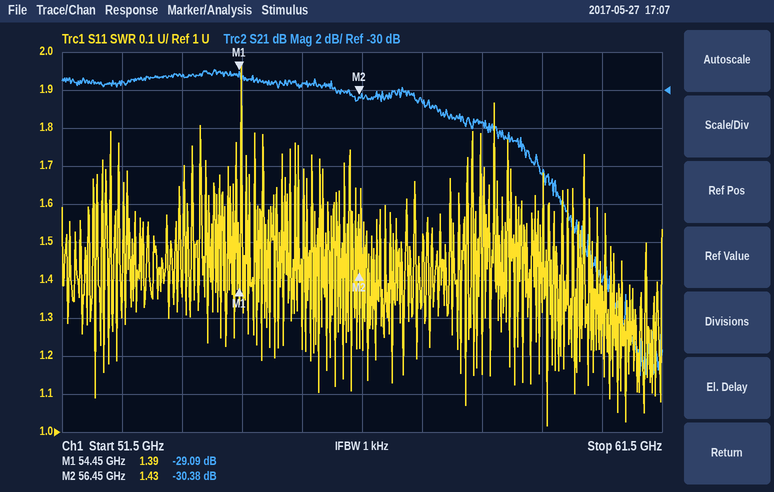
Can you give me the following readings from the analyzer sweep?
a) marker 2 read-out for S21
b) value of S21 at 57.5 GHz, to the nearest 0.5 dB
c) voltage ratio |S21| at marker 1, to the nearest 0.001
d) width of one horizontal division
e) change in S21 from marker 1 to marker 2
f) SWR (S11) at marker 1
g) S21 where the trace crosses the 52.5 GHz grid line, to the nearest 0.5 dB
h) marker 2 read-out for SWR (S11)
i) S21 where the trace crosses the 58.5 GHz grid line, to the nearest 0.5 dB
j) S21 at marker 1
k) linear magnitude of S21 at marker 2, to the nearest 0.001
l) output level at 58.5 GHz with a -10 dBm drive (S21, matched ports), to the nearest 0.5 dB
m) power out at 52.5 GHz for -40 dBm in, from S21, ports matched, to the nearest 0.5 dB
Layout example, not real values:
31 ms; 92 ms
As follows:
-30.38 dB; -30.5 dB; 0.035; 1 GHz; -1.29 dB; 1.39; -29.5 dB; 1.43; -31.5 dB; -29.09 dB; 0.030; -41.5 dBm; -69.5 dBm
